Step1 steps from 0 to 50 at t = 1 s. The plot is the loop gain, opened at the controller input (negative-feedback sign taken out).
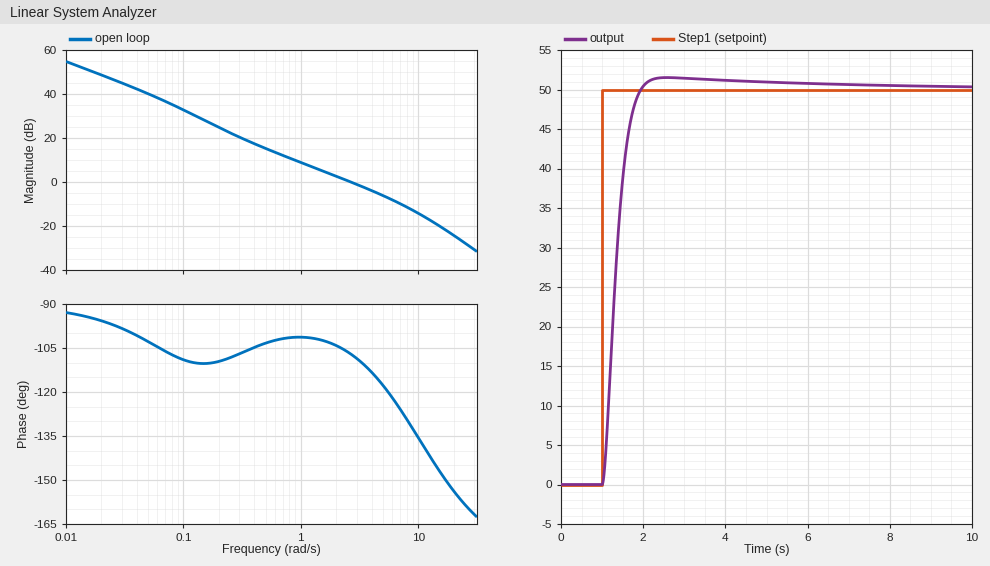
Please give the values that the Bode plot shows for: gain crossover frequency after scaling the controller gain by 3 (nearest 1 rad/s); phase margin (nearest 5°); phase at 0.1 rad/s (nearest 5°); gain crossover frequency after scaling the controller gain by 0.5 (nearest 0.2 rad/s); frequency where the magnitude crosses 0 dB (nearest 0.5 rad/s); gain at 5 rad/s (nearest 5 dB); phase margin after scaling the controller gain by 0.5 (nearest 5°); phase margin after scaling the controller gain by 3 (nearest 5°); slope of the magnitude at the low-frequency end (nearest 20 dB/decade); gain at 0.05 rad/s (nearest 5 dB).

7 rad/s
75°
-110°
1.4 rad/s
2.5 rad/s
-5 dB
80°
55°
-20 dB/decade
40 dB
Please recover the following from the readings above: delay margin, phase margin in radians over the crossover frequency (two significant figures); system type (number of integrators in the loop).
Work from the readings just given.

0.52 s
1
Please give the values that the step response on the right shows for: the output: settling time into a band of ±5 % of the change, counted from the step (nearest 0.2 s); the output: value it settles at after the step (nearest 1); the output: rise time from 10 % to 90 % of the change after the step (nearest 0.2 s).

0.8 s
50
0.6 s
